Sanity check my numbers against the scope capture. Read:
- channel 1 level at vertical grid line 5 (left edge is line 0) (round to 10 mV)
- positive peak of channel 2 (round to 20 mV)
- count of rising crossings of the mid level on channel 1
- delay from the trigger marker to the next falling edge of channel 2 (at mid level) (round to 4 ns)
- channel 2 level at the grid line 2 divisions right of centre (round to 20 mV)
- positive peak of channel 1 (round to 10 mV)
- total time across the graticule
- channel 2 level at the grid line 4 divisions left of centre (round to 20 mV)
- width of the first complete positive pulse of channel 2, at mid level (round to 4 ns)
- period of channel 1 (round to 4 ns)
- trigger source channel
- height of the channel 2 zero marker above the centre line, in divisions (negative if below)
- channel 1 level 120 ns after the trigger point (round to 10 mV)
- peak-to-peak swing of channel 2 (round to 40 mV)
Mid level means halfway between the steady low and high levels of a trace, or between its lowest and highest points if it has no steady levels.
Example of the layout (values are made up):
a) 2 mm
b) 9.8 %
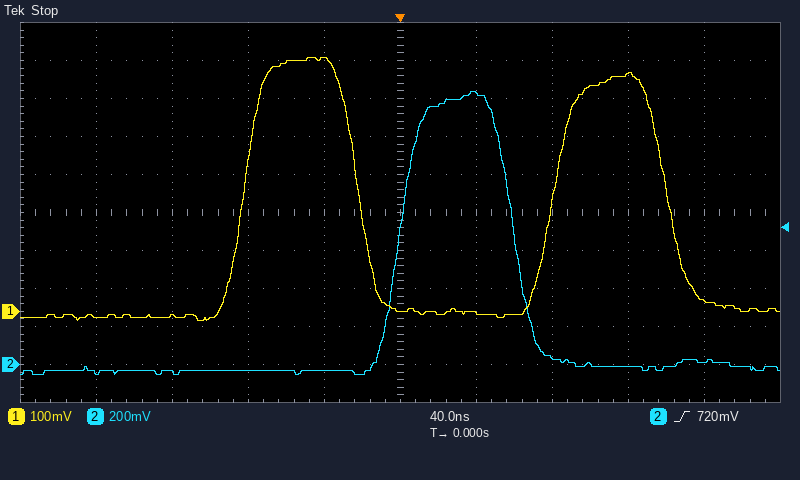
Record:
a) 0 mV
b) 1.44 V
c) 2
d) 60 ns
e) 40 mV
f) 670 mV
g) 400 ns
h) -40 mV
i) 60 ns
j) 164 ns
k) channel 2
l) -4.0 div
m) 620 mV
n) 1.48 V
